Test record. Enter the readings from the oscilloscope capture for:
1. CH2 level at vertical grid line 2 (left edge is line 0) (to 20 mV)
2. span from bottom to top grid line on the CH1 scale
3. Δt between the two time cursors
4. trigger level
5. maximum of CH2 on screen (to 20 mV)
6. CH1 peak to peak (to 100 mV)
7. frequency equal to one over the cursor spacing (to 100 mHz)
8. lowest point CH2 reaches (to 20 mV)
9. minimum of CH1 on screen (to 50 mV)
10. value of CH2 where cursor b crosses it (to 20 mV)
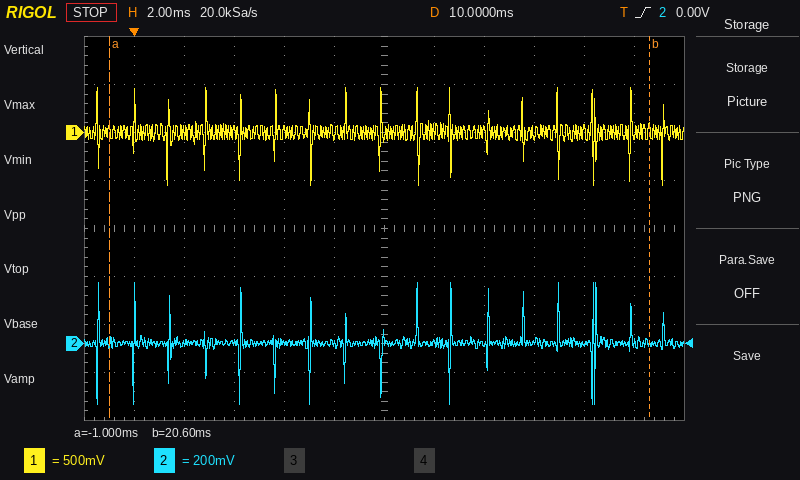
0 mV
4 V
21.6 ms
0.00 V
260 mV
1.00 V
46.3 Hz
-260 mV
-550 mV
0 mV
